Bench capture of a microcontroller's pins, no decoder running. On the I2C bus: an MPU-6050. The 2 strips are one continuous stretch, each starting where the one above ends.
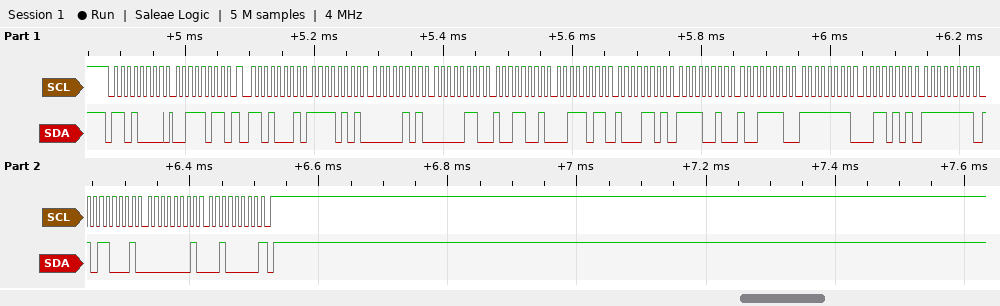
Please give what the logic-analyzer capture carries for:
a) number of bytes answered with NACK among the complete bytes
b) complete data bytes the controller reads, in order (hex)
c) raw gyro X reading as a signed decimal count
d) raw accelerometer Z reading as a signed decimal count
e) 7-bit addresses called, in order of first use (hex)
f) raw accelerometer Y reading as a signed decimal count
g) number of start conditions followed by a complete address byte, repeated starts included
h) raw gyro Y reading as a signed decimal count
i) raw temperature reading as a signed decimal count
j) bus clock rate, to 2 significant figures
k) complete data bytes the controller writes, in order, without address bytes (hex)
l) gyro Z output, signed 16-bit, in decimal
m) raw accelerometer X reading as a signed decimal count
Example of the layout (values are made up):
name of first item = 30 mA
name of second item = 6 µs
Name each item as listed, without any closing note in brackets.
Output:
number of bytes answered with NACK among the complete bytes = 1
complete data bytes the controller reads, in order = F5 05 06 99 3B 8D F2 9E FF 35 FF B1 01 20
raw gyro X reading as a signed decimal count = -203
raw accelerometer Z reading as a signed decimal count = 15245
7-bit addresses called, in order of first use = 0x68
raw accelerometer Y reading as a signed decimal count = 1689
number of start conditions followed by a complete address byte, repeated starts included = 2
raw gyro Y reading as a signed decimal count = -79
raw temperature reading as a signed decimal count = -3426
bus clock rate, to 2 significant figures = 100 kHz
complete data bytes the controller writes, in order, without address bytes = 3B
gyro Z output, signed 16-bit, in decimal = 288
raw accelerometer X reading as a signed decimal count = -2811
